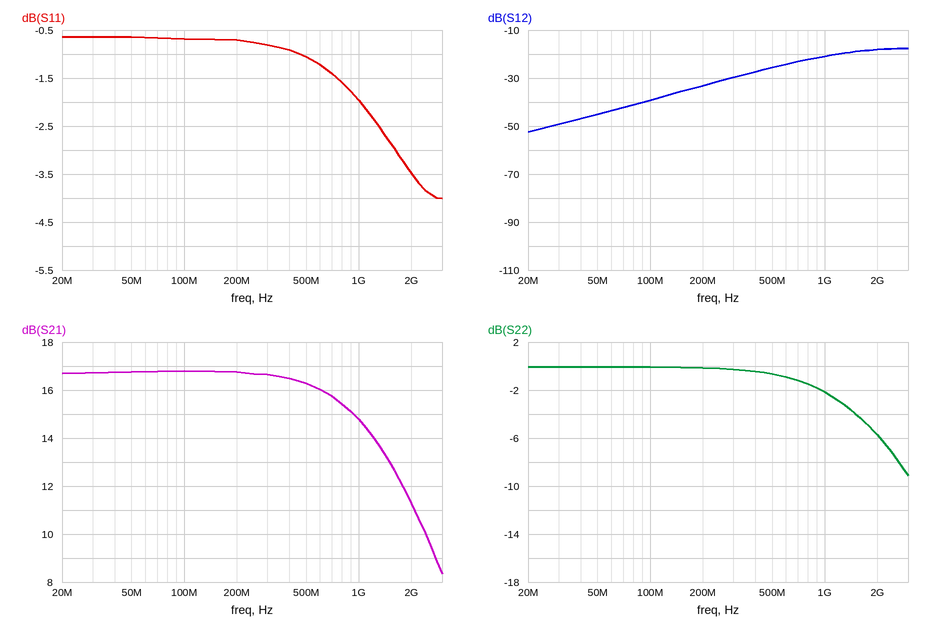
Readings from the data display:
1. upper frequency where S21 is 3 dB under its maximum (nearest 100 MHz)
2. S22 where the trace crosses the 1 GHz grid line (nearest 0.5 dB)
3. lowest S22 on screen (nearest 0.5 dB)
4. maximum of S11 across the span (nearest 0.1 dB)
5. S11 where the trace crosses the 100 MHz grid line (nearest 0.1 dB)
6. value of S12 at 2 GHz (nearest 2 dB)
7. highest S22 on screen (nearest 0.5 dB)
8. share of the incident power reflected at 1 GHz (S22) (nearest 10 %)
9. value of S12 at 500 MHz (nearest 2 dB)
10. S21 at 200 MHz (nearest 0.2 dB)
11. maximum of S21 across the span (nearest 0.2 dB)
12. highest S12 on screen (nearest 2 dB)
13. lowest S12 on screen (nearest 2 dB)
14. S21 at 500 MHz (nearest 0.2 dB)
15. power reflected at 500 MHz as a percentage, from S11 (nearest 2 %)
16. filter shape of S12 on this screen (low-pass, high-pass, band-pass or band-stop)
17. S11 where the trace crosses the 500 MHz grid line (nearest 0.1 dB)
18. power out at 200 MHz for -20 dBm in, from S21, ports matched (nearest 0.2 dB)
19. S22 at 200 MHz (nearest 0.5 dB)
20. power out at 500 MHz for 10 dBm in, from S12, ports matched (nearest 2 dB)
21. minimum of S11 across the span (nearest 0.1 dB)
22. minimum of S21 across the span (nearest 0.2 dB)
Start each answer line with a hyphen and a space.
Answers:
- 1.3 GHz
- -2.0 dB
- -9.0 dB
- -0.6 dB
- -0.7 dB
- -18 dB
- 0.0 dB
- 60 %
- -26 dB
- 16.8 dB
- 16.8 dB
- -18 dB
- -52 dB
- 16.2 dB
- 78 %
- high-pass
- -1.1 dB
- -3.2 dBm
- 0.0 dB
- -16 dBm
- -4.0 dB
- 8.4 dB
